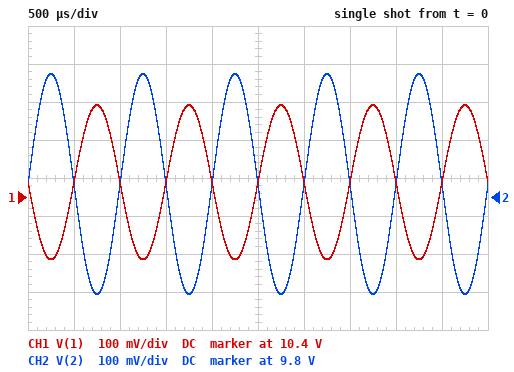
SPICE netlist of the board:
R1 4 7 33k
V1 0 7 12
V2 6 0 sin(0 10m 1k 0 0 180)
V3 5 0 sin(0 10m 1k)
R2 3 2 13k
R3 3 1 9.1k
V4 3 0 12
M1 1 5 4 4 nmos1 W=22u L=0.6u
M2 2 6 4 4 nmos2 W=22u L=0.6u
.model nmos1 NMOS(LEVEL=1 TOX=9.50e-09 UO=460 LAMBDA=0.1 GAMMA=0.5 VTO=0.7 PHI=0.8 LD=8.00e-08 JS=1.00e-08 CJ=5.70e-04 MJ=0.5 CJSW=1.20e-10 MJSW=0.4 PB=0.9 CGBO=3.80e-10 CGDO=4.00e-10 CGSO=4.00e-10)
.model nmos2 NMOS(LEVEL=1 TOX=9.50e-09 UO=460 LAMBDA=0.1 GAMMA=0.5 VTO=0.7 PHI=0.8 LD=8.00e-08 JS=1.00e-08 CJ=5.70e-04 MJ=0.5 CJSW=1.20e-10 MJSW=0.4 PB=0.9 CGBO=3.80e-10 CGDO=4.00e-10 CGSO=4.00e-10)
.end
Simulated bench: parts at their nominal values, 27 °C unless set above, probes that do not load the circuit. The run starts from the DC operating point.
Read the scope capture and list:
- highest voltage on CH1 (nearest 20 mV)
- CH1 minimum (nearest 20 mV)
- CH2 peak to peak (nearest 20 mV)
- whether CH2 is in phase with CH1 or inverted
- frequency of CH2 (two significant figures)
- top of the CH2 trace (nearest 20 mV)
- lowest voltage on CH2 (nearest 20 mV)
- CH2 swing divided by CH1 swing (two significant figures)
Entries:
10.64 V
10.24 V
580 mV
inverted
1.0 kHz
10.12 V
9.54 V
1.4
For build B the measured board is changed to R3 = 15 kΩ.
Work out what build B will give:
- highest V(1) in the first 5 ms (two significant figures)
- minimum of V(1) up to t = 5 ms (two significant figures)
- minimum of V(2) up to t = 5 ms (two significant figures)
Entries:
9.8 V
9.2 V
9.5 V
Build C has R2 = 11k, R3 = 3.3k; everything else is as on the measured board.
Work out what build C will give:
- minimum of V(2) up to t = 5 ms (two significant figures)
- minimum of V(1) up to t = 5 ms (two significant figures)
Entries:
9.9 V
11 V
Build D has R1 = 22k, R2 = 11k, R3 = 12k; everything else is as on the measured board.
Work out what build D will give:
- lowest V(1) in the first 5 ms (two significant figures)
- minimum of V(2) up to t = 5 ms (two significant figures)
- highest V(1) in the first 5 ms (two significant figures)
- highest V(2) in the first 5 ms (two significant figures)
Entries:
8.7 V
8.9 V
9.3 V
9.5 V
